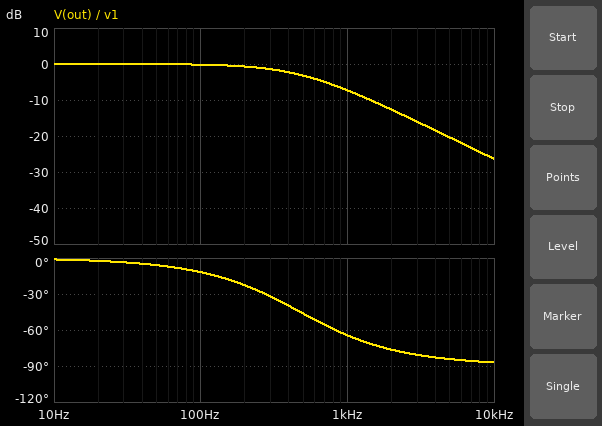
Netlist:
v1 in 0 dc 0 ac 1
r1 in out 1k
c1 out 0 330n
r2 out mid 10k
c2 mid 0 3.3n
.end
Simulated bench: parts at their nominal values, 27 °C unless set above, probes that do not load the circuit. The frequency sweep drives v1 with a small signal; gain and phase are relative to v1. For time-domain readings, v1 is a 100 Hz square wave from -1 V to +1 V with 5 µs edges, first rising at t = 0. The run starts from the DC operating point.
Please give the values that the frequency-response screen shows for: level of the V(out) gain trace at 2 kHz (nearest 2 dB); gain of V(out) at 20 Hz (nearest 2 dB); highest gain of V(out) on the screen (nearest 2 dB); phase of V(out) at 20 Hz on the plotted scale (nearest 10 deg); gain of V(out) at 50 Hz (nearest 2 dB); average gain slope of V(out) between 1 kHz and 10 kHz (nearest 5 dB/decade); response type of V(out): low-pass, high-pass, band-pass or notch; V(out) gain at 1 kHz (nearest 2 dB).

-12 dB
0 dB
0 dB
0 deg
0 dB
-20 dB/decade
low-pass
-8 dB
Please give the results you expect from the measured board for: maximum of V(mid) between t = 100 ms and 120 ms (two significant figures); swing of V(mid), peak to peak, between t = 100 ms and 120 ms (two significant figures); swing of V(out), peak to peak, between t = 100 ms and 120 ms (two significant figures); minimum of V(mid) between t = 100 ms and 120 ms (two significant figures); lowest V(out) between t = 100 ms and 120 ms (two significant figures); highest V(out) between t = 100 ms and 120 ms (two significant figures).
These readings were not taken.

1.0 V
2.0 V
2.0 V
-1.0 V
-1.0 V
1.0 V
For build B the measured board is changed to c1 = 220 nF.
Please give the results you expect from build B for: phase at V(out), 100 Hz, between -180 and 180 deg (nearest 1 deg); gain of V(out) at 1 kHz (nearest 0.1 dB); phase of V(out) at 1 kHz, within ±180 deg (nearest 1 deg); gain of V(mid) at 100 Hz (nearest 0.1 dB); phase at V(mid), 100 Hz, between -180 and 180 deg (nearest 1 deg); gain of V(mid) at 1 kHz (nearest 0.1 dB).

-8 deg
-4.7 dB
-54 deg
-0.1 dB
-9 deg
-4.9 dB
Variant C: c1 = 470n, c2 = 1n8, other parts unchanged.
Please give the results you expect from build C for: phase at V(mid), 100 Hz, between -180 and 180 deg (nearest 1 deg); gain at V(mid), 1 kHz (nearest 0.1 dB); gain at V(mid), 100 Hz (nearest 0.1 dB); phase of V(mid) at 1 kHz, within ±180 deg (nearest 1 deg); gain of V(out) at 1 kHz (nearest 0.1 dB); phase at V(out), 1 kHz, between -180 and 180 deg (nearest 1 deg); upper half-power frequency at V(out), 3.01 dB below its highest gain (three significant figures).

-17 deg
-10.0 dB
-0.4 dB
-78 deg
-9.9 dB
-71 deg
337 Hz
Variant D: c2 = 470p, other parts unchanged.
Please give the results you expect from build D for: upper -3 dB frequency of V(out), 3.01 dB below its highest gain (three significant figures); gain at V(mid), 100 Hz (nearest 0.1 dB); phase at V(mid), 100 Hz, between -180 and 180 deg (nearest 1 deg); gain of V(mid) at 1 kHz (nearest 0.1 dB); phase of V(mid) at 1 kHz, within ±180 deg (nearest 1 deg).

482 Hz
-0.2 dB
-12 deg
-7.3 dB
-66 deg
